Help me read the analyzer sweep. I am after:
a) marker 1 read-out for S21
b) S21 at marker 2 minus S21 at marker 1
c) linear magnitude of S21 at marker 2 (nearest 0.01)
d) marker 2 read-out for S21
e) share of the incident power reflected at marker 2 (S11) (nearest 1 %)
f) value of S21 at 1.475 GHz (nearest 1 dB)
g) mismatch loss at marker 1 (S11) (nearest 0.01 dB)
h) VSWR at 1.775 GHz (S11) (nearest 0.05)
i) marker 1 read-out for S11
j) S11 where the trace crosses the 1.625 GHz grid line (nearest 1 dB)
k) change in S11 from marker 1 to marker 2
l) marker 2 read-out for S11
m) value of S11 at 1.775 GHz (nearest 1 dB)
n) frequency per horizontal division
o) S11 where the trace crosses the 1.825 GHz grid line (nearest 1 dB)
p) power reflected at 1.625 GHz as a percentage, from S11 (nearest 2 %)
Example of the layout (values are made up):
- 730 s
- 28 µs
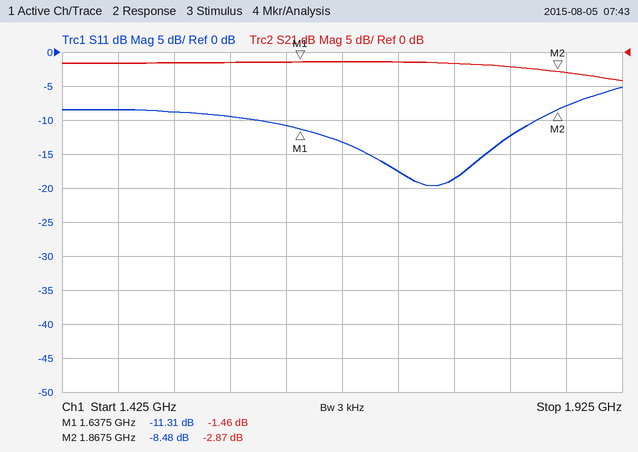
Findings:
- -1.46 dB
- -1.41 dB
- 0.72
- -2.87 dB
- 14 %
- -2 dB
- 0.33 dB
- 1.25
- -11.31 dB
- -11 dB
- 2.83 dB
- -8.48 dB
- -19 dB
- 50 MHz
- -12 dB
- 8 %
